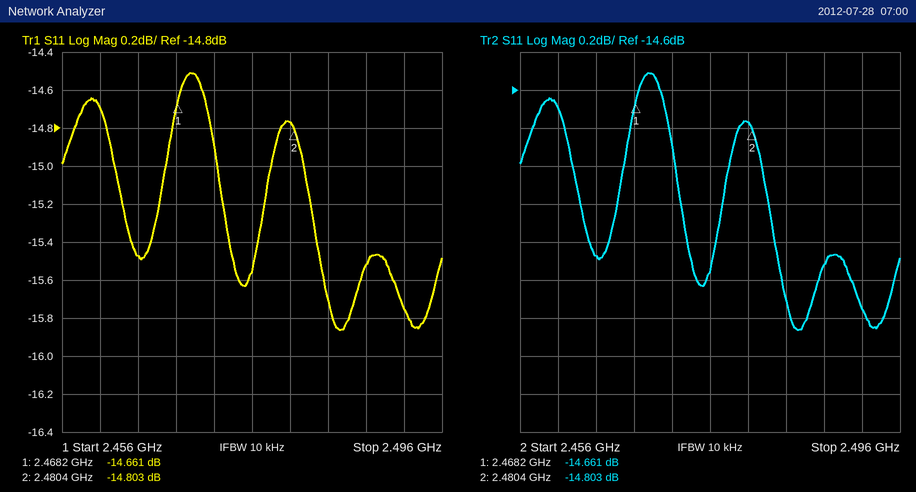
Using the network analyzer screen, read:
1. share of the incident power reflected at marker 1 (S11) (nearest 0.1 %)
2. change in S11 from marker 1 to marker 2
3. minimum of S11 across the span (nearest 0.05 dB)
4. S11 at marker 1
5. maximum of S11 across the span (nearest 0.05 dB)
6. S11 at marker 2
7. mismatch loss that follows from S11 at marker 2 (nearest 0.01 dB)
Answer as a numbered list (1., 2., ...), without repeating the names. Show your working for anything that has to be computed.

1. 10^(-14.661/10) ≈ 3.4 %
2. -14.803 − (-14.661) = -0.142 dB
3. -15.85 dB
4. -14.661 dB
5. -14.50 dB
6. -14.803 dB
7. −10 log10(1 − 10^(-14.803/10)) ≈ 0.15 dB
